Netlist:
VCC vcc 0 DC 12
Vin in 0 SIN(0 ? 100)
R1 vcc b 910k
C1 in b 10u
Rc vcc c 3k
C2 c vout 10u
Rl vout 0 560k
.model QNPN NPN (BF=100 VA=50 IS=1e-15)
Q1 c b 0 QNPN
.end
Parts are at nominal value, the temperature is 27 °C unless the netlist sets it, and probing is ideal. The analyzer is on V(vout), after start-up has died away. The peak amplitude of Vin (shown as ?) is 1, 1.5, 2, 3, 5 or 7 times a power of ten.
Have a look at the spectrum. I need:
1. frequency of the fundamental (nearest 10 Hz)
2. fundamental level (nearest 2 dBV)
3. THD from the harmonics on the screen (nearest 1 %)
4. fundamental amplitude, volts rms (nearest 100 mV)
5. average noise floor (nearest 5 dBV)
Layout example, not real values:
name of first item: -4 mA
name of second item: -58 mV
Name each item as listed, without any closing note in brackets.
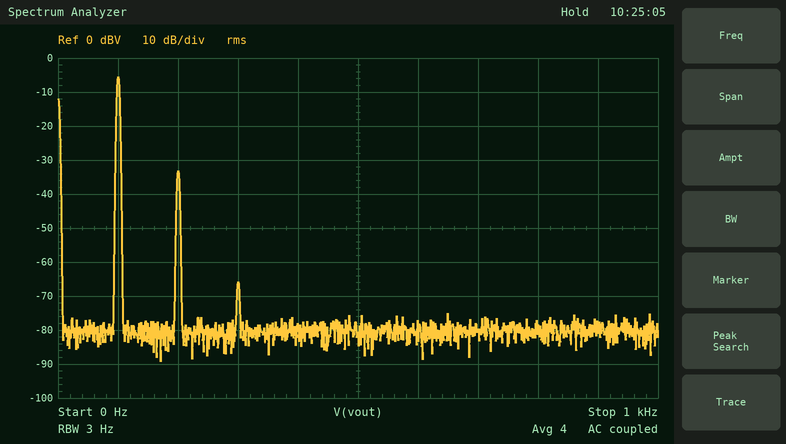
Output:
frequency of the fundamental: 100 Hz
fundamental level: -6 dBV
THD from the harmonics on the screen: 4 %
fundamental amplitude, volts rms: 500 mV
average noise floor: -80 dBV
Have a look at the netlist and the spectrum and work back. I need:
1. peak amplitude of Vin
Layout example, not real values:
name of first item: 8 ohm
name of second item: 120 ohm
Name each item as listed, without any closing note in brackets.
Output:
peak amplitude of Vin: 5 mV
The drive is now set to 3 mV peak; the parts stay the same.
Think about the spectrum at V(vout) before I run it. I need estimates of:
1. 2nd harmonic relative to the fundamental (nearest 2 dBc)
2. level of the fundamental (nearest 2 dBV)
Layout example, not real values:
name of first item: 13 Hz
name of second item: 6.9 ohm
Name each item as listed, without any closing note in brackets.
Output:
2nd harmonic relative to the fundamental: -32 dBc
level of the fundamental: -10 dBV
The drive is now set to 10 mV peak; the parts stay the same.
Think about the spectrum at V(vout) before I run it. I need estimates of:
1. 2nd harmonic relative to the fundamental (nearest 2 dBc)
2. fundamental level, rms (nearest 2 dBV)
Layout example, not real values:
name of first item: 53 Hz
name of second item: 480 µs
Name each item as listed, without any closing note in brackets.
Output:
2nd harmonic relative to the fundamental: -22 dBc
fundamental level, rms: 0 dBV
